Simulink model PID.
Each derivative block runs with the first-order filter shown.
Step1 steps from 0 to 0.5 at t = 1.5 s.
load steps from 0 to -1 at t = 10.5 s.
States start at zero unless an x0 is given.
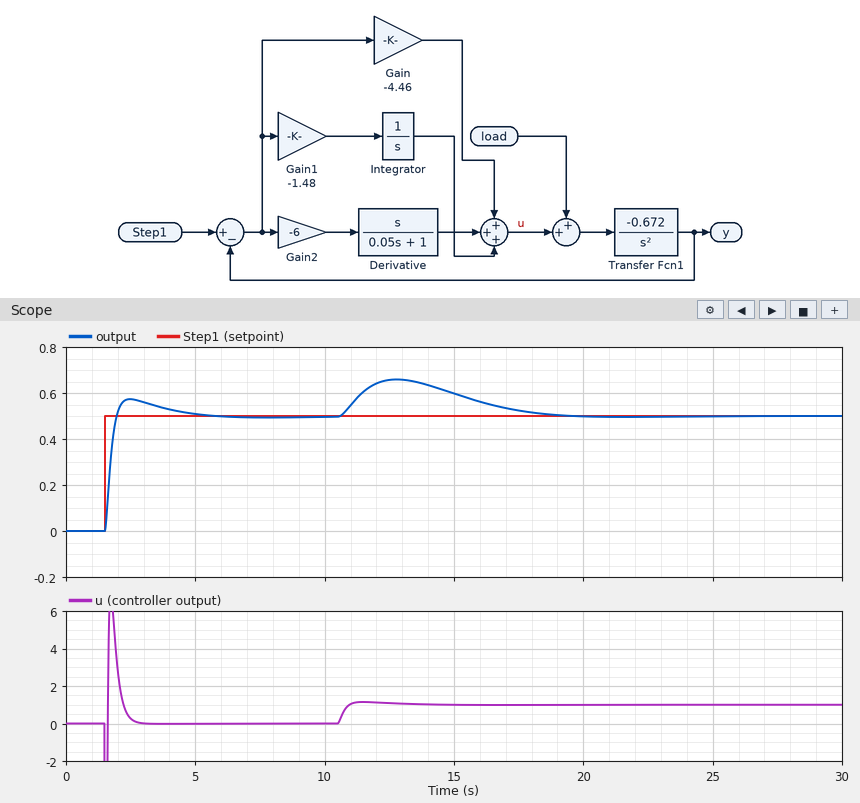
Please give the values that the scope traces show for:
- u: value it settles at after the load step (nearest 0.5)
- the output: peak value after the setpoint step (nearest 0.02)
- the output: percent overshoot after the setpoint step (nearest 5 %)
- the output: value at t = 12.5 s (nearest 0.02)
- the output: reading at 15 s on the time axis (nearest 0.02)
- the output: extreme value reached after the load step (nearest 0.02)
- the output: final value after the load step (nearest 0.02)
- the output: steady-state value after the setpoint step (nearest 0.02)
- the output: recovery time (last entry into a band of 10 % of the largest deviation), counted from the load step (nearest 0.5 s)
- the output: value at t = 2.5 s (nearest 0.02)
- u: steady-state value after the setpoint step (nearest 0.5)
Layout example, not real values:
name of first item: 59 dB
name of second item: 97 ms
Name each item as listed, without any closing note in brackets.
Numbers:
u: value it settles at after the load step: 1.0
the output: peak value after the setpoint step: 0.58
the output: percent overshoot after the setpoint step: 15 %
the output: value at t = 12.5 s: 0.66
the output: reading at 15 s on the time axis: 0.60
the output: extreme value reached after the load step: 0.66
the output: final value after the load step: 0.50
the output: steady-state value after the setpoint step: 0.50
the output: recovery time (last entry into a band of 10 % of the largest deviation), counted from the load step: 7.5 s
the output: value at t = 2.5 s: 0.58
u: steady-state value after the setpoint step: 0.0
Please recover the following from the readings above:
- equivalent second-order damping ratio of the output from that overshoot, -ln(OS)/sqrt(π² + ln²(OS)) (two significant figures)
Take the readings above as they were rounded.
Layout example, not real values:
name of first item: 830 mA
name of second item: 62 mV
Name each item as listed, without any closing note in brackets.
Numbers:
equivalent second-order damping ratio of the output from that overshoot, -ln(OS)/sqrt(π² + ln²(OS)): 0.52
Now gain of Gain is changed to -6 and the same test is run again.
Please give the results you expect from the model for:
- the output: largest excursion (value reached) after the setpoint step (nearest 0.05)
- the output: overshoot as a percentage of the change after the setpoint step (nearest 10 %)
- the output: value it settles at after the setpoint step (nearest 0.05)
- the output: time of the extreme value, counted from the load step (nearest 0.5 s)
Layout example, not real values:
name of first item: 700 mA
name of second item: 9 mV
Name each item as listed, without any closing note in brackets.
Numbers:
the output: largest excursion (value reached) after the setpoint step: 0.60
the output: overshoot as a percentage of the change after the setpoint step: 20 %
the output: value it settles at after the setpoint step: 0.50
the output: time of the extreme value, counted from the load step: 2.0 s
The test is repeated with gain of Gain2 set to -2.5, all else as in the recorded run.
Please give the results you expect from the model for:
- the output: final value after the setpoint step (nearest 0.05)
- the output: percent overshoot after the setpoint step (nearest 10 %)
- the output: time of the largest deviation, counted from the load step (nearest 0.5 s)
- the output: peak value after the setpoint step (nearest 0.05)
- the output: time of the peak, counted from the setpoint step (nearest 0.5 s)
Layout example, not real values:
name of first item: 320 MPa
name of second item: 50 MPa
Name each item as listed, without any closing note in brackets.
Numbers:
the output: final value after the setpoint step: 0.50
the output: percent overshoot after the setpoint step: 40 %
the output: time of the largest deviation, counted from the load step: 1.5 s
the output: peak value after the setpoint step: 0.70
the output: time of the peak, counted from the setpoint step: 1.5 s
